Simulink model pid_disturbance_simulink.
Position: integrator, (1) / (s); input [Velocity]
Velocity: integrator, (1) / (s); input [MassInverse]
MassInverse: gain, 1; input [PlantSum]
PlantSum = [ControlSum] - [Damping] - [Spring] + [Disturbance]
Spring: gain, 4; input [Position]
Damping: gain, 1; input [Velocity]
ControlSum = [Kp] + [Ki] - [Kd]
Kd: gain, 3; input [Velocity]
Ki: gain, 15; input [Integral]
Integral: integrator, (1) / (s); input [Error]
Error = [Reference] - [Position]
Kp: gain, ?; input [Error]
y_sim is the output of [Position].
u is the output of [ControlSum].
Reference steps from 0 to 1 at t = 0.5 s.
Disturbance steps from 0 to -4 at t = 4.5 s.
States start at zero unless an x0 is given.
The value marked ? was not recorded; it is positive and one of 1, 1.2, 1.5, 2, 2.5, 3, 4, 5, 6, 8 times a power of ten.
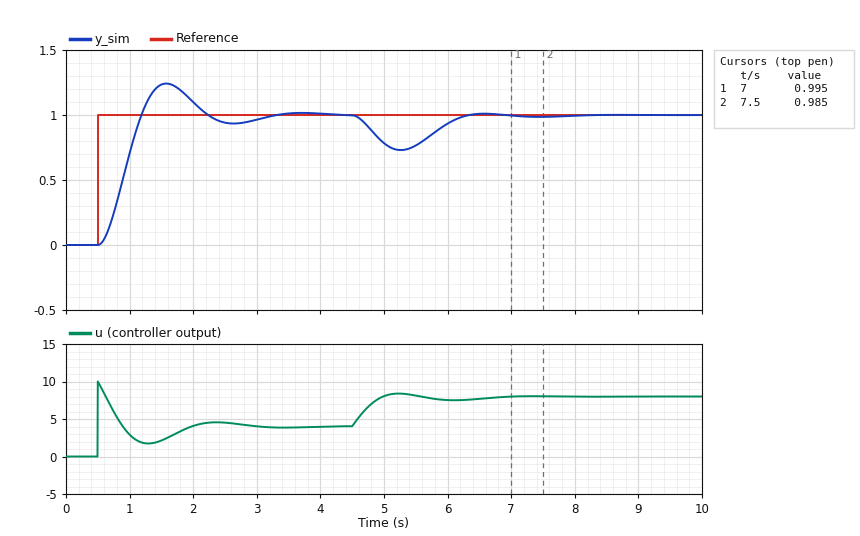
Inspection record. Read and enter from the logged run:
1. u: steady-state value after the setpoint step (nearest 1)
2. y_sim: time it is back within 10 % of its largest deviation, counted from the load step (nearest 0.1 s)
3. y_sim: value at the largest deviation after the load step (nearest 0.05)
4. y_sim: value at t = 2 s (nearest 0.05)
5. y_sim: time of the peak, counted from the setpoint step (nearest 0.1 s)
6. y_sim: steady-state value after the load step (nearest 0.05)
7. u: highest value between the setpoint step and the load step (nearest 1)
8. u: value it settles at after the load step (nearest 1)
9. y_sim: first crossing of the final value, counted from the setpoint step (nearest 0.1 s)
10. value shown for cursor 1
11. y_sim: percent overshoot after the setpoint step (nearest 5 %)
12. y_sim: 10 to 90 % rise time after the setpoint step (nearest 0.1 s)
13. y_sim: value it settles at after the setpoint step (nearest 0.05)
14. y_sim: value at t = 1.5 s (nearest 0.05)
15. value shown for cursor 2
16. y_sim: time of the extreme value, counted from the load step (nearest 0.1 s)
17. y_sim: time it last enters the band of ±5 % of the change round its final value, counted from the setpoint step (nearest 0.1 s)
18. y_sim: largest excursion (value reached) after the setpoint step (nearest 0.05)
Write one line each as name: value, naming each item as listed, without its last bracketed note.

u: steady-state value after the setpoint step: 4
y_sim: time it is back within 10 % of its largest deviation, counted from the load step: 1.7 s
y_sim: value at the largest deviation after the load step: 0.75
y_sim: value at t = 2 s: 1.10
y_sim: time of the peak, counted from the setpoint step: 1.1 s
y_sim: steady-state value after the load step: 1.00
u: highest value between the setpoint step and the load step: 10
u: value it settles at after the load step: 8
y_sim: first crossing of the final value, counted from the setpoint step: 0.7 s
value shown for cursor 1: 0.995
y_sim: percent overshoot after the setpoint step: 25 %
y_sim: 10 to 90 % rise time after the setpoint step: 0.5 s
y_sim: value it settles at after the setpoint step: 1.00
y_sim: value at t = 1.5 s: 1.25
value shown for cursor 2: 0.985
y_sim: time of the extreme value, counted from the load step: 0.8 s
y_sim: time it last enters the band of ±5 % of the change round its final value, counted from the setpoint step: 2.4 s
y_sim: largest excursion (value reached) after the setpoint step: 1.25
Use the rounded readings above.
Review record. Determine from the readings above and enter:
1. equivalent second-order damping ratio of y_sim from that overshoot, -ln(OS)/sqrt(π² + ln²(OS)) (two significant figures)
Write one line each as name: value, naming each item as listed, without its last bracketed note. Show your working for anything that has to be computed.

equivalent second-order damping ratio of y_sim from that overshoot, -ln(OS)/sqrt(π² + ln²(OS)): ln(0.25) = -1.386; 1.386 / sqrt(9.870 + 1.922) = 0.40
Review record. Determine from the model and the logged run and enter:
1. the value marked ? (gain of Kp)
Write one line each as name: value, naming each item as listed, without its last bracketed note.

the value marked ?: 10
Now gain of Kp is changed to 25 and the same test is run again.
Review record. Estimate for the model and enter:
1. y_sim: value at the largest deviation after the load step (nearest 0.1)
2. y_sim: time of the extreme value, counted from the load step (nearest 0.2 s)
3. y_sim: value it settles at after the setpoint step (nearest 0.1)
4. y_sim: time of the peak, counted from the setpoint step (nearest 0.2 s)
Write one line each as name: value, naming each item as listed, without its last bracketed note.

y_sim: value at the largest deviation after the load step: 0.8
y_sim: time of the extreme value, counted from the load step: 0.6 s
y_sim: value it settles at after the setpoint step: 1.0
y_sim: time of the peak, counted from the setpoint step: 0.6 s
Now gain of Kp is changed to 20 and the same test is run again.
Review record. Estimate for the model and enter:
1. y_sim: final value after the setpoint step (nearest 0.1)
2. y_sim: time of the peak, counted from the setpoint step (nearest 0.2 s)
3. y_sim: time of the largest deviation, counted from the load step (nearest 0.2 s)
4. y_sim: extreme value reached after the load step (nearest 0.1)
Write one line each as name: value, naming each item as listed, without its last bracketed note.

y_sim: final value after the setpoint step: 1.0
y_sim: time of the peak, counted from the setpoint step: 0.8 s
y_sim: time of the largest deviation, counted from the load step: 0.6 s
y_sim: extreme value reached after the load step: 0.8
